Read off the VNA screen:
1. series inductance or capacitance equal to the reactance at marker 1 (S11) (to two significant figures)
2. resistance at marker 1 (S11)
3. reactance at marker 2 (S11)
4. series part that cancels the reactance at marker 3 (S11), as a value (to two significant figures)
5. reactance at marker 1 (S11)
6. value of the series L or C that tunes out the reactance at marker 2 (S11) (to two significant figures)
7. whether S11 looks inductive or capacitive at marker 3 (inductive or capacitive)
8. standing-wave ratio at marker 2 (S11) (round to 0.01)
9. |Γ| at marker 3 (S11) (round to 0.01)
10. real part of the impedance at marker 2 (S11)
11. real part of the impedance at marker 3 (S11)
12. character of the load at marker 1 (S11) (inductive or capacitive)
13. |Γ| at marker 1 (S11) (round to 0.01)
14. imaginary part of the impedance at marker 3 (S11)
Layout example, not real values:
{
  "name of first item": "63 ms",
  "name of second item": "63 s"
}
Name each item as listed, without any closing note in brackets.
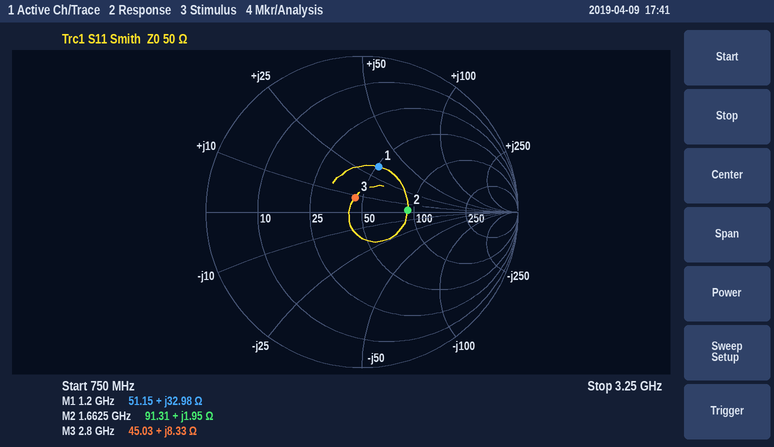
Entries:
{
  "series inductance or capacitance equal to the reactance at marker 1 (S11)": "4.4 nH",
  "resistance at marker 1": "51.15 Ω",
  "reactance at marker 2": "+1.95 Ω",
  "series part that cancels the reactance at marker 3 (S11), as a value": "6.8 pF",
  "reactance at marker 1": "+32.98 Ω",
  "value of the series L or C that tunes out the reactance at marker 2 (S11)": "49 pF",
  "whether S11 looks inductive or capacitive at marker 3": "inductive",
  "standing-wave ratio at marker 2 (S11)": "1.83",
  "|Γ| at marker 3 (S11)": "0.10",
  "real part of the impedance at marker 2": "91.31 Ω",
  "real part of the impedance at marker 3": "45.03 Ω",
  "character of the load at marker 1 (S11)": "inductive",
  "|Γ| at marker 1 (S11)": "0.31",
  "imaginary part of the impedance at marker 3": "+8.33 Ω"
}
